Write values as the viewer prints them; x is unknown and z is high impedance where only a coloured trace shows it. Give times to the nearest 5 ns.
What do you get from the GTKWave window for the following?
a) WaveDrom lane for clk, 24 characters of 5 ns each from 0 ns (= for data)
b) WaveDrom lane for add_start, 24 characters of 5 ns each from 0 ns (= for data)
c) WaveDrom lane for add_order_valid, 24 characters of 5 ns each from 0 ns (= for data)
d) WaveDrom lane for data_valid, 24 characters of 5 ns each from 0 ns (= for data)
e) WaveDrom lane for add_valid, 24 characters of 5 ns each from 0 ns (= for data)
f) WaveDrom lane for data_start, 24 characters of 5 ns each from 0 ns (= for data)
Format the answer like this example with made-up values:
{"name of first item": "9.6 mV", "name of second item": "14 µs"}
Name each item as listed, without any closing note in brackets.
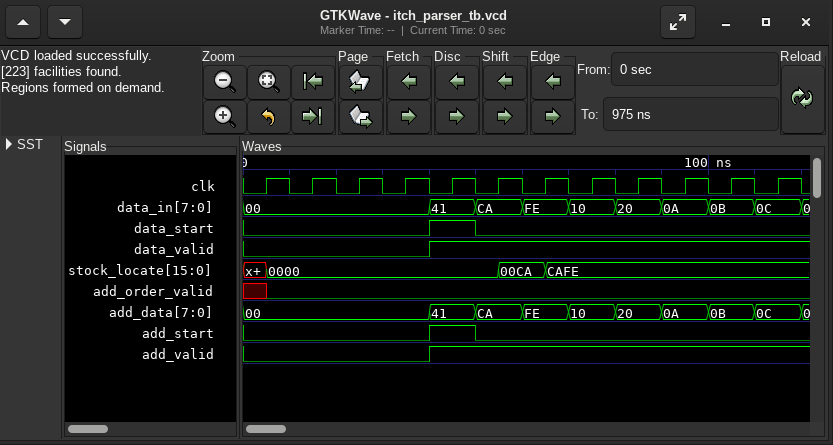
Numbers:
{"WaveDrom lane for clk, 24 characters of 5 ns each from 0 ns": "{name: 'clk', wave: '010101010101010101010101'}", "WaveDrom lane for add_start, 24 characters of 5 ns each from 0 ns": "{name: 'add_start', wave: '0.......1.0.............'}", "WaveDrom lane for add_order_valid, 24 characters of 5 ns each from 0 ns": "{name: 'add_order_valid', wave: 'x0......................'}", "WaveDrom lane for data_valid, 24 characters of 5 ns each from 0 ns": "{name: 'data_valid', wave: '0.......1...............'}", "WaveDrom lane for add_valid, 24 characters of 5 ns each from 0 ns": "{name: 'add_valid', wave: '0.......1...............'}", "WaveDrom lane for data_start, 24 characters of 5 ns each from 0 ns": "{name: 'data_start', wave: '0.......1.0.............'}"}
